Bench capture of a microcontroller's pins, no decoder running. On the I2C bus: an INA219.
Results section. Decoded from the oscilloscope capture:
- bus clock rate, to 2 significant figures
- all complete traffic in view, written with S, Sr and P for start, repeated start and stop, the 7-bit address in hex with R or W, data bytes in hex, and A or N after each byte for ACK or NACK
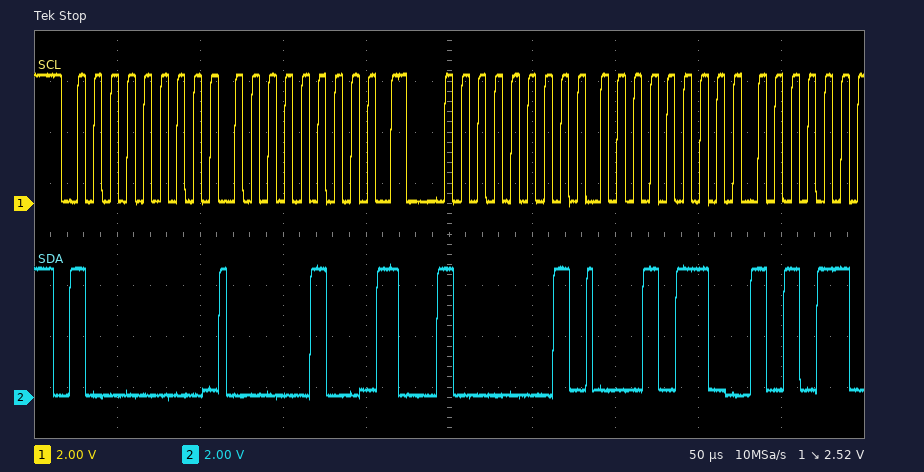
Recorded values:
100 kHz
S 40W A 04 A Sr 40R A 16 A
